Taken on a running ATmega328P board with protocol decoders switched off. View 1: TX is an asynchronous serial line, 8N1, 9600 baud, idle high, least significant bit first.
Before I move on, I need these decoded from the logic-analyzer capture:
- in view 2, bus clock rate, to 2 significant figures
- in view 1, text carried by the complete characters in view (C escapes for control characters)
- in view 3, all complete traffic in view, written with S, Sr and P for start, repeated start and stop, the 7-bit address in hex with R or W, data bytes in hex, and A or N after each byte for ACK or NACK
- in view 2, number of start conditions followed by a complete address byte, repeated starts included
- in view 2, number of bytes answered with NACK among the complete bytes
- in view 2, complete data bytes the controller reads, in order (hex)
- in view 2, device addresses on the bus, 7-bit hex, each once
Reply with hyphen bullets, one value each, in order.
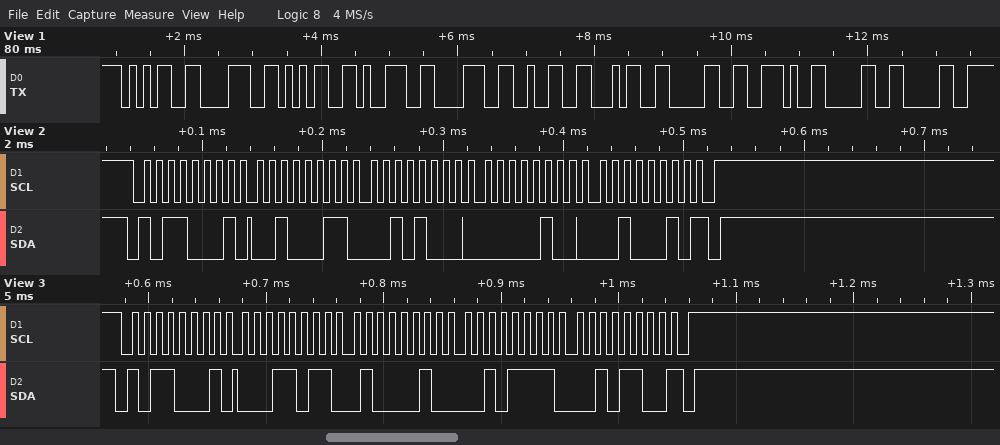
- 100 kHz
- "58598240.00"
- S 58R A 1B A 42 A 2F A 2C N P
- 1
- 1
- 23 28 04 22
- 0x58
